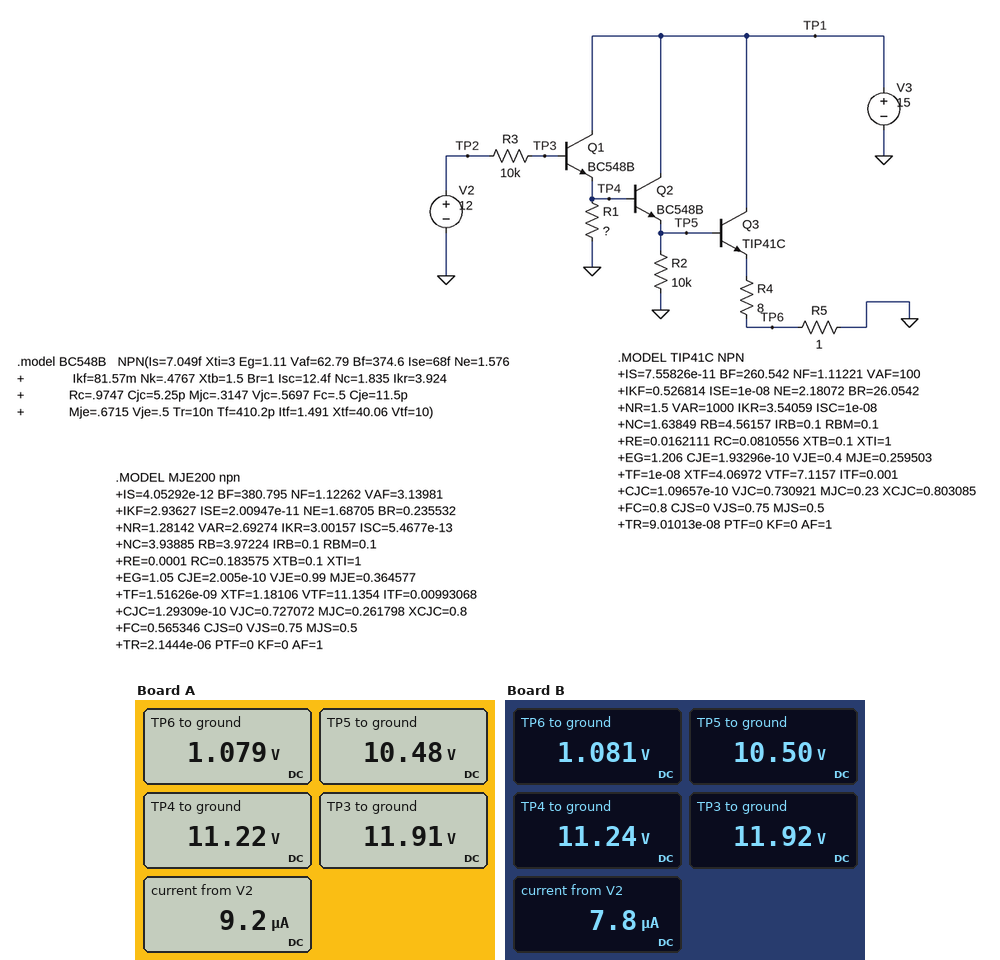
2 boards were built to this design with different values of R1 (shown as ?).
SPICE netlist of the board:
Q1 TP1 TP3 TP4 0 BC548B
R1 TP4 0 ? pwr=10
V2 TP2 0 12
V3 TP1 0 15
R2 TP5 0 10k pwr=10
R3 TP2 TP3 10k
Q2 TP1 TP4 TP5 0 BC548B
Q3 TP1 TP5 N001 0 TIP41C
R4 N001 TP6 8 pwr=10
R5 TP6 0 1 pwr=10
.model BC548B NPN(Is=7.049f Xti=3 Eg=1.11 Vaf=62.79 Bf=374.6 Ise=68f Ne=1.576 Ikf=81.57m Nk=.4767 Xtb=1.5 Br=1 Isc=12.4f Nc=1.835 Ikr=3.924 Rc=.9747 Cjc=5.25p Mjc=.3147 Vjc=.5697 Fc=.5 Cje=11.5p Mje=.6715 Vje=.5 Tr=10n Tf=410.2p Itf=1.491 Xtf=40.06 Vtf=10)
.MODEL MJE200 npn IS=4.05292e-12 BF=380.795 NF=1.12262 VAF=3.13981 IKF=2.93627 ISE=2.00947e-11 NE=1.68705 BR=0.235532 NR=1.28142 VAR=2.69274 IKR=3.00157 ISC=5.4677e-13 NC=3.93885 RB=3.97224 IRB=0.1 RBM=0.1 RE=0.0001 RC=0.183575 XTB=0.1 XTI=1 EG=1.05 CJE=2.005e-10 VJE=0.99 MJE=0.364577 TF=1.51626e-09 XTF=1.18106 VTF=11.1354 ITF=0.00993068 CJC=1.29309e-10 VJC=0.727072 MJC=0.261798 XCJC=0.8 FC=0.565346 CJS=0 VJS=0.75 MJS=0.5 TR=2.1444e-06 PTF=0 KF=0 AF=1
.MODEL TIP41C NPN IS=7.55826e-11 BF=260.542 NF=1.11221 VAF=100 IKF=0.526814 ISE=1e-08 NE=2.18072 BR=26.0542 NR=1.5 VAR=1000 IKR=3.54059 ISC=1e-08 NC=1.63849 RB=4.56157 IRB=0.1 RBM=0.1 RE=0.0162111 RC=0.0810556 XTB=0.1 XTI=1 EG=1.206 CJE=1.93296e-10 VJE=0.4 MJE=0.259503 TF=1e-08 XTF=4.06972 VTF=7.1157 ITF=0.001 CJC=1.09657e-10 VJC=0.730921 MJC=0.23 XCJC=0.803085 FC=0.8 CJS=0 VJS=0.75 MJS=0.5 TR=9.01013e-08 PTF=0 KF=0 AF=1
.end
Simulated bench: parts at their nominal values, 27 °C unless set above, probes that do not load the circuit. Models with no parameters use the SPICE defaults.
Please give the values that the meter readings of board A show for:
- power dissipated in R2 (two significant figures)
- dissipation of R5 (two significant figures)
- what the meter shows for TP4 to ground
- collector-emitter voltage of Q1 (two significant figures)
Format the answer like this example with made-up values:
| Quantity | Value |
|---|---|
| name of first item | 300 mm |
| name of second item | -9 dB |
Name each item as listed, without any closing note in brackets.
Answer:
| Quantity | Value |
|---|---|
| power dissipated in R2 | 11 mW |
| dissipation of R5 | 1.2 W |
| what the meter shows for TP4 to ground | 11.22 V |
| collector-emitter voltage of Q1 | 3.8 V |
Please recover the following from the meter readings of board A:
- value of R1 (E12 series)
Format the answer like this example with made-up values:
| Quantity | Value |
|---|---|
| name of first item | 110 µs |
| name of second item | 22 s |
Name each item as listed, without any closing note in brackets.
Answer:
| Quantity | Value |
|---|---|
| value of R1 | 3.9 kΩ |
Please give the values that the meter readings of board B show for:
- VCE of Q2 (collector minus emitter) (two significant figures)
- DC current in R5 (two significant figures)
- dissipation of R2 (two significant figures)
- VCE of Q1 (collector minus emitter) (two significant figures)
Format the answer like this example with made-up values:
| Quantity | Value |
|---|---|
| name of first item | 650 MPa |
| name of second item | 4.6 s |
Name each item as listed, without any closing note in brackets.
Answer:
| Quantity | Value |
|---|---|
| VCE of Q2 (collector minus emitter) | 4.5 V |
| DC current in R5 | 1.1 A |
| dissipation of R2 | 11 mW |
| VCE of Q1 (collector minus emitter) | 3.8 V |
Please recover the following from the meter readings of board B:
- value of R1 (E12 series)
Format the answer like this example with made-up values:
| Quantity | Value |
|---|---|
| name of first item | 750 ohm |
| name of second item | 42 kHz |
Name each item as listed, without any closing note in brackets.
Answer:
| Quantity | Value |
|---|---|
| value of R1 | 4.7 kΩ |
